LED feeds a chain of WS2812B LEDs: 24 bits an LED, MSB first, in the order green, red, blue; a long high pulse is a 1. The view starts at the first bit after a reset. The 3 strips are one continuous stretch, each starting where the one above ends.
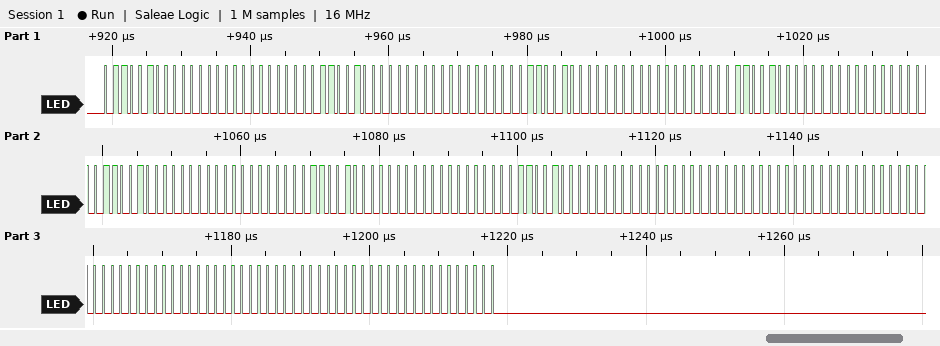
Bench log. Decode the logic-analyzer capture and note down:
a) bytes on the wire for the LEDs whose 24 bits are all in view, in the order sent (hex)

64 00 00 64 00 00 64 00 00 64 00 00 64 00 00 64 00 00 64 00 00 00 00 00 00 00 00 00 00 00
